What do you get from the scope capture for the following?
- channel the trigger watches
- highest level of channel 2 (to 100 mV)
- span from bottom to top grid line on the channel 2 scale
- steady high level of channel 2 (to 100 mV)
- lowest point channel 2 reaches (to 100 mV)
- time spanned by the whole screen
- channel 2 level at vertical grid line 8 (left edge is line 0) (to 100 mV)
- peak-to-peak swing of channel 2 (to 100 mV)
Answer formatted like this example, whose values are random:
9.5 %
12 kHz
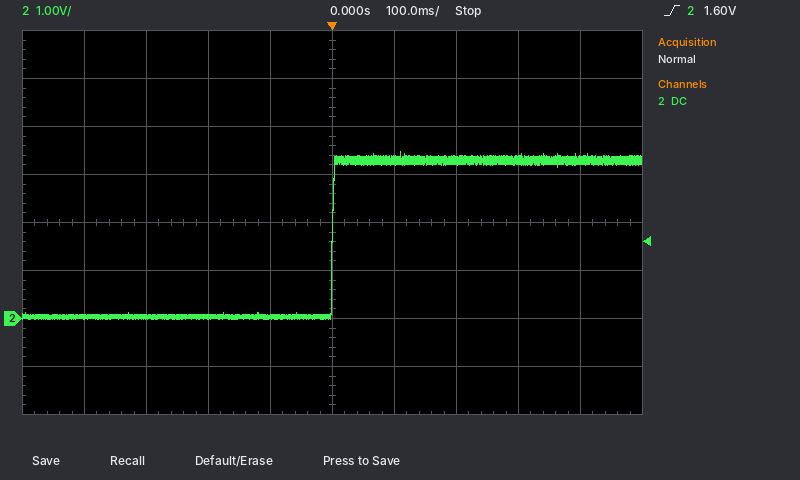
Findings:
channel 2
3.5 V
8 V
3.3 V
0.0 V
1 s
3.3 V
3.5 V
